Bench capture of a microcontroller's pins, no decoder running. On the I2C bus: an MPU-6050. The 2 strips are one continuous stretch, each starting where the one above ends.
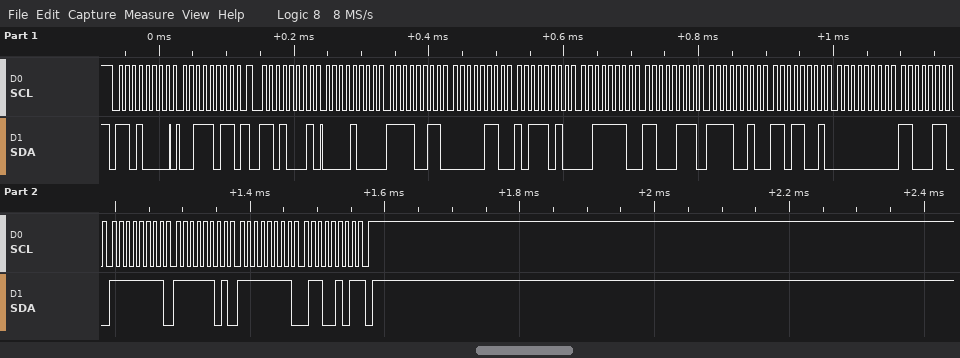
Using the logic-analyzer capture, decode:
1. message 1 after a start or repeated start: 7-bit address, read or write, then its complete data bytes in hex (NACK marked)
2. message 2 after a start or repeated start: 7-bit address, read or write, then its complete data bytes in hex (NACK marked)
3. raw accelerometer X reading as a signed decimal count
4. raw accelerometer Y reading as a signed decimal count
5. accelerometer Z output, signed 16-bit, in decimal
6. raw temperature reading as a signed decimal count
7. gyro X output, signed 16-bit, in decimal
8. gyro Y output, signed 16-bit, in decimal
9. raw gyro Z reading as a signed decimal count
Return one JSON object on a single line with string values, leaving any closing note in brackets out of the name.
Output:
{"message 1 after a start or repeated start: 7-bit address, read or write, then its complete data bytes in hex": "0x68 write: 3B", "message 2 after a start or repeated start: 7-bit address, read or write, then its complete data bytes in hex": "0x68 read: 08 F3 06 BA 3E C7 F2 D9 00 C6 FF FD FF 65 NACK", "raw accelerometer X reading as a signed decimal count": "2291", "raw accelerometer Y reading as a signed decimal count": "1722", "accelerometer Z output, signed 16-bit, in decimal": "16071", "raw temperature reading as a signed decimal count": "-3367", "gyro X output, signed 16-bit, in decimal": "198", "gyro Y output, signed 16-bit, in decimal": "-3", "raw gyro Z reading as a signed decimal count": "-155"}
